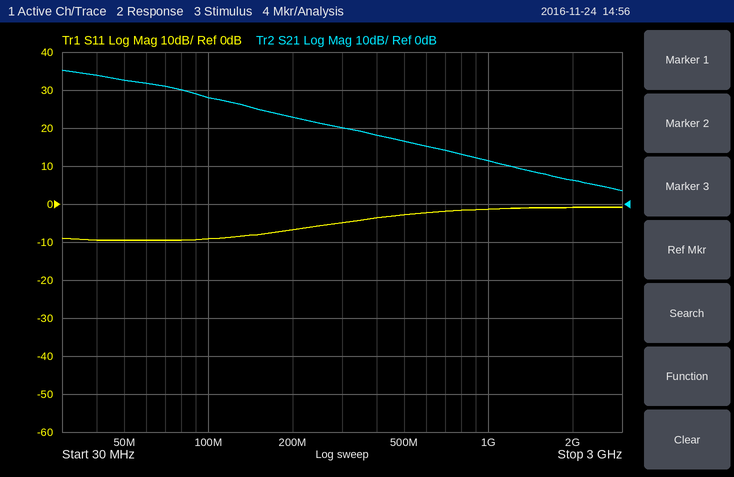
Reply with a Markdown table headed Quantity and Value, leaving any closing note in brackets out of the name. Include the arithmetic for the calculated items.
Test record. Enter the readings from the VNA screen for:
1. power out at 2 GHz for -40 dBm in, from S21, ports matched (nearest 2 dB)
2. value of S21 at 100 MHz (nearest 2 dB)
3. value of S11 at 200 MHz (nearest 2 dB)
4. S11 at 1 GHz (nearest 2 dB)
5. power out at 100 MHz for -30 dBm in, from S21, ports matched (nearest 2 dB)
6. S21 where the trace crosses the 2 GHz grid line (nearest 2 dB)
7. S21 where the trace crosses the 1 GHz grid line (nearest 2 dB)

| Quantity | Value |
|---|---|
| power out at 2 GHz for -40 dBm in, from S21, ports matched | -40 dBm + (6 dB) = -34 dBm |
| value of S21 at 100 MHz | 28 dB |
| value of S11 at 200 MHz | -6 dB |
| S11 at 1 GHz | -2 dB |
| power out at 100 MHz for -30 dBm in, from S21, ports matched | -30 dBm + (28 dB) = -2 dBm |
| S21 where the trace crosses the 2 GHz grid line | 6 dB |
| S21 where the trace crosses the 1 GHz grid line | 12 dB |
